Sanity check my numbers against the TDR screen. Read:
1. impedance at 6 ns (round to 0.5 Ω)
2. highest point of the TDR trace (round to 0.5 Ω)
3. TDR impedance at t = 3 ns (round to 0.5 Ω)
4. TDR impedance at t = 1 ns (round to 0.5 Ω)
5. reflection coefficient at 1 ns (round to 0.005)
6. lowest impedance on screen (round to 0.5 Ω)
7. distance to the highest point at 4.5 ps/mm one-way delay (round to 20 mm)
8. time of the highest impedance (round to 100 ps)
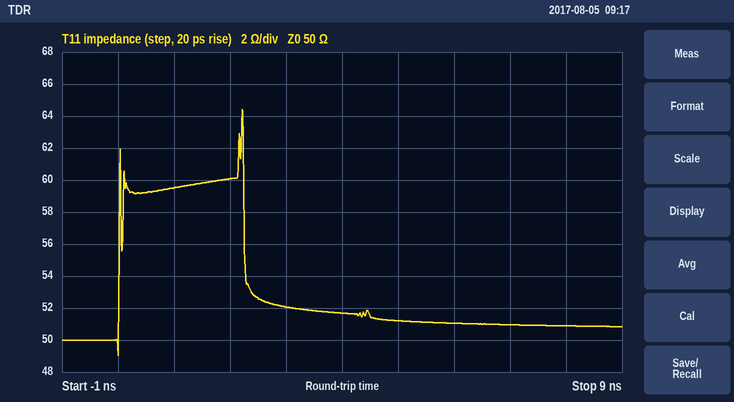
51.0 Ω
64.5 Ω
52.0 Ω
59.5 Ω
+0.085
49.0 Ω
240 mm
2.2 ns
